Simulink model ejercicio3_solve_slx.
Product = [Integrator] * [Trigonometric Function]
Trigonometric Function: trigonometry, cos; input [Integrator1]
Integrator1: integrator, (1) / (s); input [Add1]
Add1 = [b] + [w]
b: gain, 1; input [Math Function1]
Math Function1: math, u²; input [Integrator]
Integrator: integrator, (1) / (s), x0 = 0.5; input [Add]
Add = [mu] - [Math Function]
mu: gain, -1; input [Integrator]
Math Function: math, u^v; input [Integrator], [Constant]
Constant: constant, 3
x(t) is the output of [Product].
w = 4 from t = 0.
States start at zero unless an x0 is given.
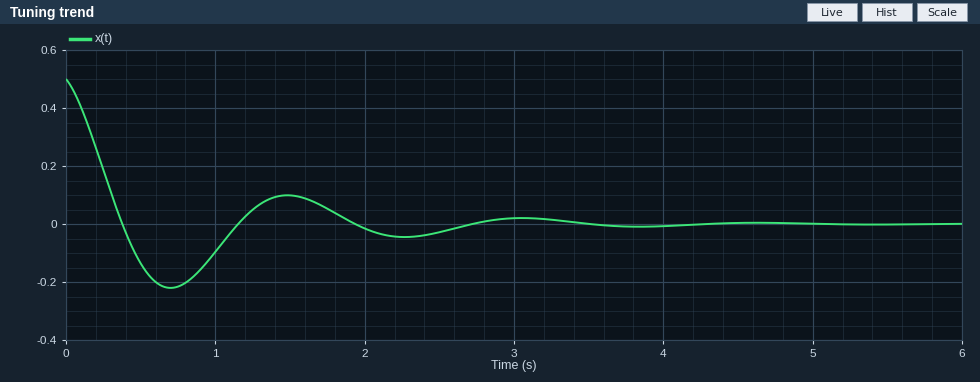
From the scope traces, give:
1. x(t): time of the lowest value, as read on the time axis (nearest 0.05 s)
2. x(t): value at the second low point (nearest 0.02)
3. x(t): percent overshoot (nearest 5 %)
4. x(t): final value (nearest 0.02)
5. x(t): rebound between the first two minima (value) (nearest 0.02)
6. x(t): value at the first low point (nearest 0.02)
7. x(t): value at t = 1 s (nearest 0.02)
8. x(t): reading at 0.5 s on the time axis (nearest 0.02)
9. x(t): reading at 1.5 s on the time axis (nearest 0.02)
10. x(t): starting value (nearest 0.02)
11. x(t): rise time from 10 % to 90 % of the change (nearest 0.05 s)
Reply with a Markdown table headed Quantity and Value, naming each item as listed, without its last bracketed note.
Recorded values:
| Quantity | Value |
|---|---|
| x(t): time of the lowest value, as read on the time axis | 0.70 s |
| x(t): value at the second low point | -0.04 |
| x(t): percent overshoot | 45 % |
| x(t): final value | 0.00 |
| x(t): rebound between the first two minima (value) | 0.10 |
| x(t): value at the first low point | -0.22 |
| x(t): value at t = 1 s | -0.10 |
| x(t): reading at 0.5 s on the time axis | -0.14 |
| x(t): reading at 1.5 s on the time axis | 0.10 |
| x(t): starting value | 0.50 |
| x(t): rise time from 10 % to 90 % of the change | 0.30 s |
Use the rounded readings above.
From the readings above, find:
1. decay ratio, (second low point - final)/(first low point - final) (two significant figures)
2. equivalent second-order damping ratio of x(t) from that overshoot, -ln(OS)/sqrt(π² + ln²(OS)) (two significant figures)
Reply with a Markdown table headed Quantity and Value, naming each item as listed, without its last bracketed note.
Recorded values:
| Quantity | Value |
|---|---|
| decay ratio, (second low point - final)/(first low point - final) | 0.18 |
| equivalent second-order damping ratio of x(t) from that overshoot, -ln(OS)/sqrt(π² + ln²(OS)) | 0.25 |
